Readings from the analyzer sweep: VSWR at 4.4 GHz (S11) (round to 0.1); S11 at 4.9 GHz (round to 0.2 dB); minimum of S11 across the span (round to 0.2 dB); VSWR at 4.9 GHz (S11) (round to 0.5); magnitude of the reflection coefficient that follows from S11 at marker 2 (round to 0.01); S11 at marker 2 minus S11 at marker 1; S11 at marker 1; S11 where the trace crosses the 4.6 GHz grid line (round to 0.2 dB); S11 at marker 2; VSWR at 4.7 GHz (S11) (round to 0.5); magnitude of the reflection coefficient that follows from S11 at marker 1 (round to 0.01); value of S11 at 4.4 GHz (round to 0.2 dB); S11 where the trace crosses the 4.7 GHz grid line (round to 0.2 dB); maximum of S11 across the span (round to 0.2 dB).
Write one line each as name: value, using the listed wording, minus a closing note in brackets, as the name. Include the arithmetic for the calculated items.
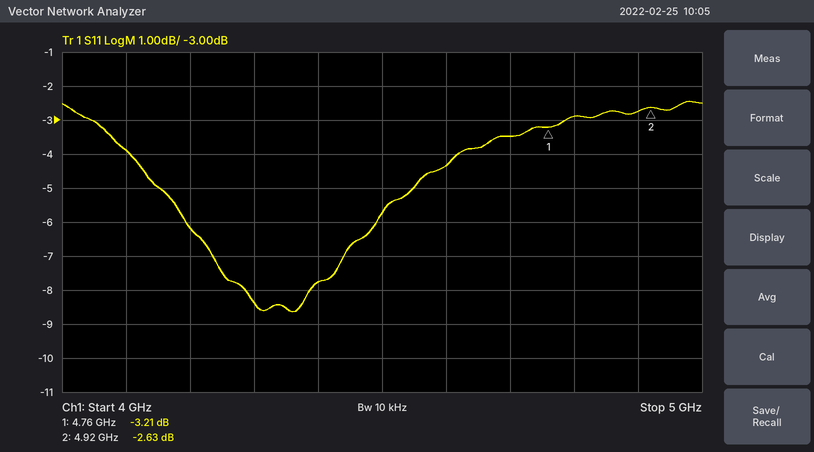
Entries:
VSWR at 4.4 GHz (S11): |Γ| = 10^(-7.8/20) = 0.4074; VSWR = (1 + 0.4074)/(1 − 0.4074) ≈ 2.4
S11 at 4.9 GHz: -2.8 dB
minimum of S11 across the span: -8.6 dB
VSWR at 4.9 GHz (S11): |Γ| = 10^(-2.8/20) = 0.7244; VSWR = (1 + 0.7244)/(1 − 0.7244) ≈ 6.26, so 6.5 to the nearest 0.5
magnitude of the reflection coefficient that follows from S11 at marker 2: 10^(-2.63/20) ≈ 0.74
S11 at marker 2 minus S11 at marker 1: -2.63 − (-3.21) = 0.58 dB
S11 at marker 1: -3.21 dB
S11 where the trace crosses the 4.6 GHz grid line: -4.4 dB
S11 at marker 2: -2.63 dB
VSWR at 4.7 GHz (S11): |Γ| = 10^(-3.4/20) = 0.6761; VSWR = (1 + 0.6761)/(1 − 0.6761) ≈ 5.17, so 5.0 to the nearest 0.5
magnitude of the reflection coefficient that follows from S11 at marker 1: 10^(-3.21/20) ≈ 0.69
value of S11 at 4.4 GHz: -7.8 dB
S11 where the trace crosses the 4.7 GHz grid line: -3.4 dB
maximum of S11 across the span: -2.4 dB
